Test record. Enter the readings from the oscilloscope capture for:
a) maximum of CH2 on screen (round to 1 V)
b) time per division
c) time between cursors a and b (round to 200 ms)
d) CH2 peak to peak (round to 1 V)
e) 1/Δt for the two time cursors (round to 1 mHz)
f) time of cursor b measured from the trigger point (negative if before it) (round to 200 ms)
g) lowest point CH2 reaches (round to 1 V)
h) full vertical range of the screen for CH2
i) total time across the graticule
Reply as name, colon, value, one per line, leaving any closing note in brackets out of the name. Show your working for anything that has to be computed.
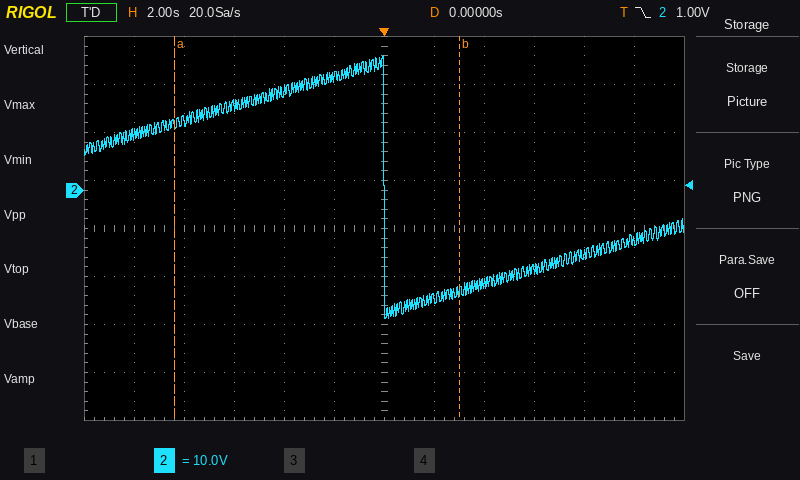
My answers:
maximum of CH2 on screen: 28 V
time per division: 2 s
time between cursors a and b: 11.4 s
CH2 peak to peak: 28 V − (-27 V) = 55 V
1/Δt for the two time cursors: 1 / 11.4 s ≈ 88 mHz
time of cursor b measured from the trigger point (negative if before it): +3.0 s
lowest point CH2 reaches: -27 V
full vertical range of the screen for CH2: 80 V
total time across the graticule: 24 s
